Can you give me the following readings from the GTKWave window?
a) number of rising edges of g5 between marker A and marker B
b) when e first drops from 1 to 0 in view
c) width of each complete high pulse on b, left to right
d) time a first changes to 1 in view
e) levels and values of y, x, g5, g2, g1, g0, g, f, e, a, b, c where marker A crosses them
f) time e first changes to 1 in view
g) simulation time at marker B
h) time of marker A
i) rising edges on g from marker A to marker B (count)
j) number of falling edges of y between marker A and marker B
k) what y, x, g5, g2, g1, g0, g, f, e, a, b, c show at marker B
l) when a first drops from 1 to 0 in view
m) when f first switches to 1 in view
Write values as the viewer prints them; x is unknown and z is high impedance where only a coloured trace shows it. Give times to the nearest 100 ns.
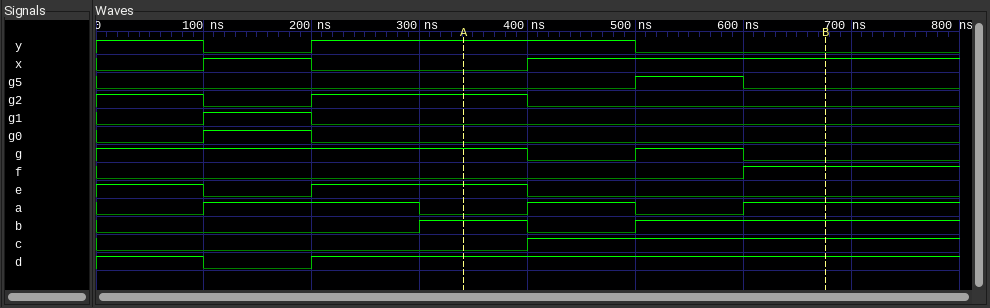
1
100 ns
100 ns
100 ns
y=1, x=0, g5=0, g2=1, g1=0, g0=0, g=1, f=0, e=1, a=0, b=1, c=0
200 ns
700 ns
300 ns
1
1
y=0, x=1, g5=0, g2=0, g1=0, g0=0, g=0, f=1, e=0, a=1, b=1, c=1
300 ns
600 ns
